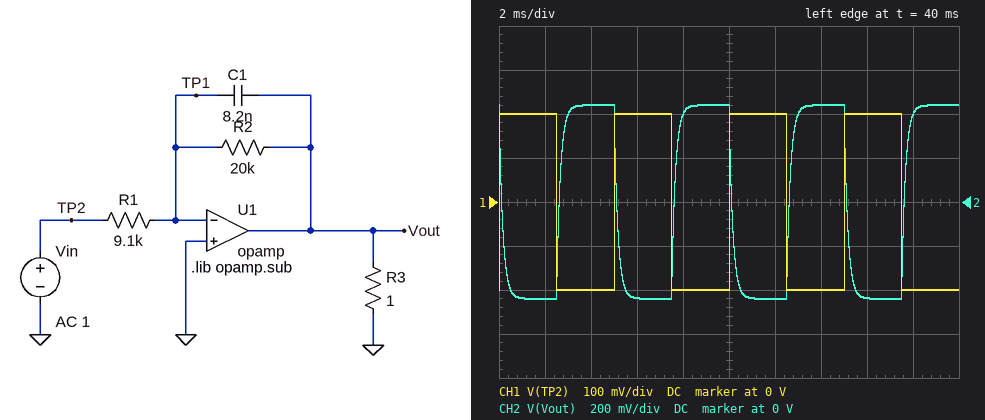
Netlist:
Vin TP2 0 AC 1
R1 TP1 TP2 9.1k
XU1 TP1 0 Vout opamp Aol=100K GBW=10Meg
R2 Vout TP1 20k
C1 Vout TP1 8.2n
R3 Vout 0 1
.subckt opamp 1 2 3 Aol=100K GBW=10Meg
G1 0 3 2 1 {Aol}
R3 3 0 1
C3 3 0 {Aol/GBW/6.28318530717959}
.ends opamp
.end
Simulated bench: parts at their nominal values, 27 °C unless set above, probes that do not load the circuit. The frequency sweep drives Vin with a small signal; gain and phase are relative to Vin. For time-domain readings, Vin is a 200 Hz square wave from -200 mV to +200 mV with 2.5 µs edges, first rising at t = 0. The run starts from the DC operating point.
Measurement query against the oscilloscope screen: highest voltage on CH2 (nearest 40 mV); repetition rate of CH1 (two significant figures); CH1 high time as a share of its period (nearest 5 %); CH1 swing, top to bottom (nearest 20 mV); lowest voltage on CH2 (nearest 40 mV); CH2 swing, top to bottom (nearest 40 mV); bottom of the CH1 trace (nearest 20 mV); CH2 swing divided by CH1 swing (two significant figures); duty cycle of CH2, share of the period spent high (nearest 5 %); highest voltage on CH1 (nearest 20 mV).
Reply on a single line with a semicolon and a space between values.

440 mV; 200 Hz; 50 %; 400 mV; -440 mV; 880 mV; -200 mV; 2.2; 50 %; 200 mV
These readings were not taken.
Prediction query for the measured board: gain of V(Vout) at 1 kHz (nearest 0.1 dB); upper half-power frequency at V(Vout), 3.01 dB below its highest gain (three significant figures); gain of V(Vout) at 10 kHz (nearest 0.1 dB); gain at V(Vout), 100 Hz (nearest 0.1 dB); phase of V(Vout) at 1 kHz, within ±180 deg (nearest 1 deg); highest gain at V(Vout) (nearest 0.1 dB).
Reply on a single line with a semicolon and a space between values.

3.7 dB; 970 Hz; -13.5 dB; 6.8 dB; 134 deg; 6.8 dB
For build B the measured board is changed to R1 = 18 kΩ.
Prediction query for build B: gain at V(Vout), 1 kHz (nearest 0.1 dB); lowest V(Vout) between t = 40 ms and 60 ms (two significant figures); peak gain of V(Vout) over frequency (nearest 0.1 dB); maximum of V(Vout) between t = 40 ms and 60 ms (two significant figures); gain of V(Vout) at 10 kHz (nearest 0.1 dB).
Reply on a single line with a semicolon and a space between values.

-2.2 dB; -220 mV; 0.9 dB; 220 mV; -19.4 dB
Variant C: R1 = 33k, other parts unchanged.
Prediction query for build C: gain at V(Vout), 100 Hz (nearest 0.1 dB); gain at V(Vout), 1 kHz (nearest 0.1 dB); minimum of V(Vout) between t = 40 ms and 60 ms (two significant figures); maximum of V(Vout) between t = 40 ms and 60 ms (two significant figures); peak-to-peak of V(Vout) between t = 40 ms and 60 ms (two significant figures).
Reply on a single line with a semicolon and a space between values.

-4.4 dB; -7.5 dB; -120 mV; 120 mV; 240 mV
